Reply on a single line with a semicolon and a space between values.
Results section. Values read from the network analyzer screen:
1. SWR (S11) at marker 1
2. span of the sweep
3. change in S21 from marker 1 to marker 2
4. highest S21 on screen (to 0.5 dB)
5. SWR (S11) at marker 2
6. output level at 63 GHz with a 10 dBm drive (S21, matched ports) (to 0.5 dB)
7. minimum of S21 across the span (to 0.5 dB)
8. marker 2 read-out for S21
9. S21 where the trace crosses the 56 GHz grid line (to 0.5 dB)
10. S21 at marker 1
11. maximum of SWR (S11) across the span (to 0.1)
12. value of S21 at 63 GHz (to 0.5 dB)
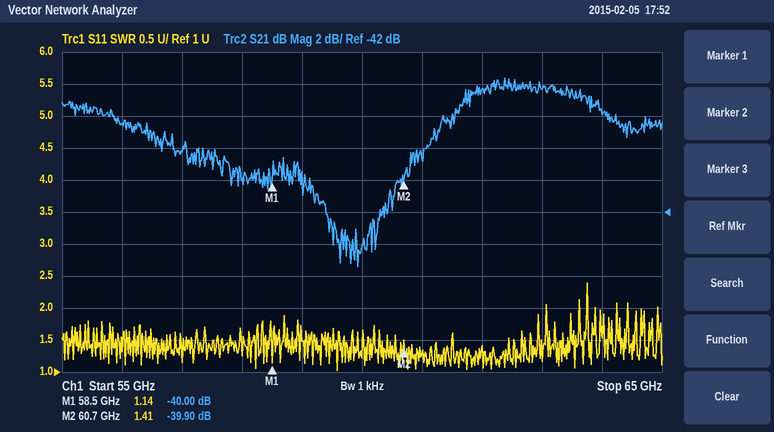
1.14; 10 GHz; 0.10 dB; -33.5 dB; 1.41; -24.5 dBm; -45.5 dB; -39.90 dB; -36.5 dB; -40.00 dB; 2.4; -34.5 dB
